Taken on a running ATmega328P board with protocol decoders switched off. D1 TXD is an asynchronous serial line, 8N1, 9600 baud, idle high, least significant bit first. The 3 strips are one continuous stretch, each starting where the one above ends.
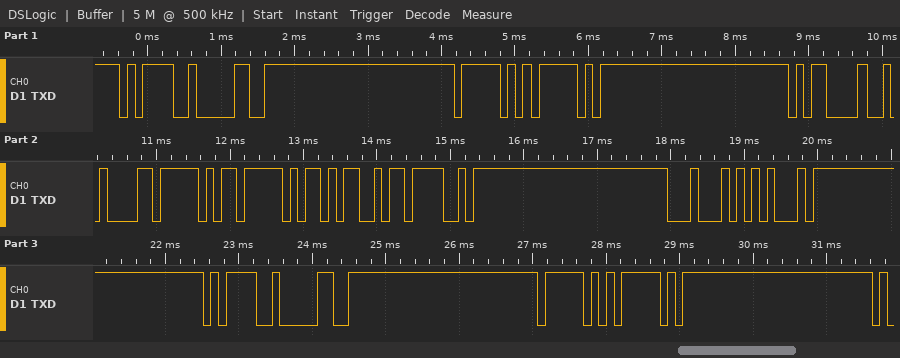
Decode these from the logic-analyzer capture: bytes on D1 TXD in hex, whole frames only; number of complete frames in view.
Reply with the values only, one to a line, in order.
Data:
0x3D 0x30 0x5F 0x5F 0x0D 0x0A 0x5F 0x5F 0x4D 0x4F 0x44 0x45 0x3D 0x30 0x5F 0x5F
16
